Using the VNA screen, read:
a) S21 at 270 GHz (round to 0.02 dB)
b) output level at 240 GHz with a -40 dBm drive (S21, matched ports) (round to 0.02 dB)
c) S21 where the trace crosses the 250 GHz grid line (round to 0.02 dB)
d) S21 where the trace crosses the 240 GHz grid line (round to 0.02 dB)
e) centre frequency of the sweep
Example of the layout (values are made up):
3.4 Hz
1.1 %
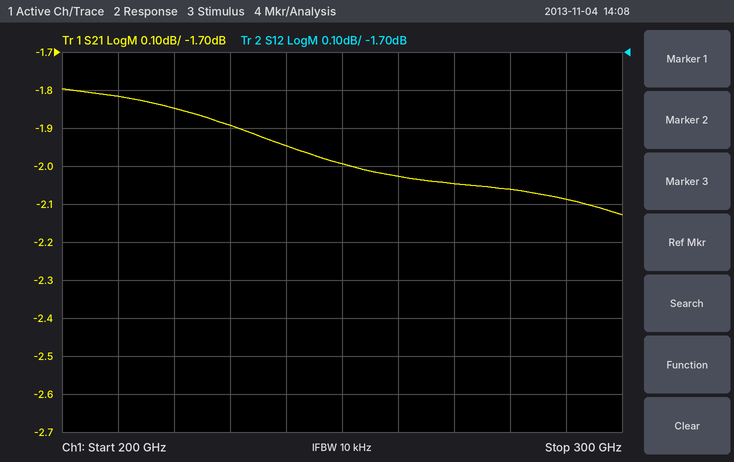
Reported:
-2.04 dB
-41.94 dBm
-2.00 dB
-1.94 dB
250 GHz
